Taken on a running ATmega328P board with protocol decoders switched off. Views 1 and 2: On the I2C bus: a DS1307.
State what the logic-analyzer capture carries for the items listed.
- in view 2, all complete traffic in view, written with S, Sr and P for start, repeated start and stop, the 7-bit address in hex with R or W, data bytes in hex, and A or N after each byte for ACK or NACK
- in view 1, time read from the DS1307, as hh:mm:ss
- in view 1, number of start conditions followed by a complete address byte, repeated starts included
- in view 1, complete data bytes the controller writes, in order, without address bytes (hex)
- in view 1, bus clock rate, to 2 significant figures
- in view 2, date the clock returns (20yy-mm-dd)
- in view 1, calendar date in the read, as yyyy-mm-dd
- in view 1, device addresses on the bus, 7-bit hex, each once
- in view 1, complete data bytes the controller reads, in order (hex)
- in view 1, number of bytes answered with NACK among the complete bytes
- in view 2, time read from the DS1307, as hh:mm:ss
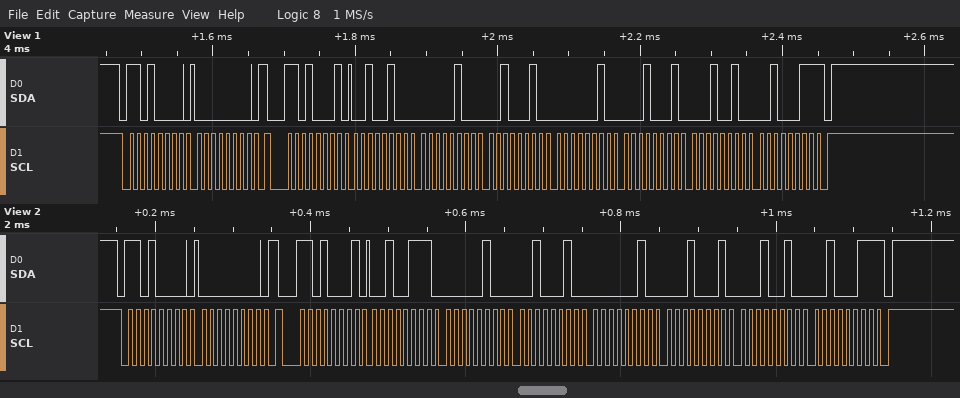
S 68W A 00 A Sr 68R A 27 A 04 A 22 A 02 A 11 A 12 A 23 N P
22:04:24
2
00
100 kHz
2023-12-11
2023-12-11
0x68
24 04 22 02 11 12 23
1
22:04:27
